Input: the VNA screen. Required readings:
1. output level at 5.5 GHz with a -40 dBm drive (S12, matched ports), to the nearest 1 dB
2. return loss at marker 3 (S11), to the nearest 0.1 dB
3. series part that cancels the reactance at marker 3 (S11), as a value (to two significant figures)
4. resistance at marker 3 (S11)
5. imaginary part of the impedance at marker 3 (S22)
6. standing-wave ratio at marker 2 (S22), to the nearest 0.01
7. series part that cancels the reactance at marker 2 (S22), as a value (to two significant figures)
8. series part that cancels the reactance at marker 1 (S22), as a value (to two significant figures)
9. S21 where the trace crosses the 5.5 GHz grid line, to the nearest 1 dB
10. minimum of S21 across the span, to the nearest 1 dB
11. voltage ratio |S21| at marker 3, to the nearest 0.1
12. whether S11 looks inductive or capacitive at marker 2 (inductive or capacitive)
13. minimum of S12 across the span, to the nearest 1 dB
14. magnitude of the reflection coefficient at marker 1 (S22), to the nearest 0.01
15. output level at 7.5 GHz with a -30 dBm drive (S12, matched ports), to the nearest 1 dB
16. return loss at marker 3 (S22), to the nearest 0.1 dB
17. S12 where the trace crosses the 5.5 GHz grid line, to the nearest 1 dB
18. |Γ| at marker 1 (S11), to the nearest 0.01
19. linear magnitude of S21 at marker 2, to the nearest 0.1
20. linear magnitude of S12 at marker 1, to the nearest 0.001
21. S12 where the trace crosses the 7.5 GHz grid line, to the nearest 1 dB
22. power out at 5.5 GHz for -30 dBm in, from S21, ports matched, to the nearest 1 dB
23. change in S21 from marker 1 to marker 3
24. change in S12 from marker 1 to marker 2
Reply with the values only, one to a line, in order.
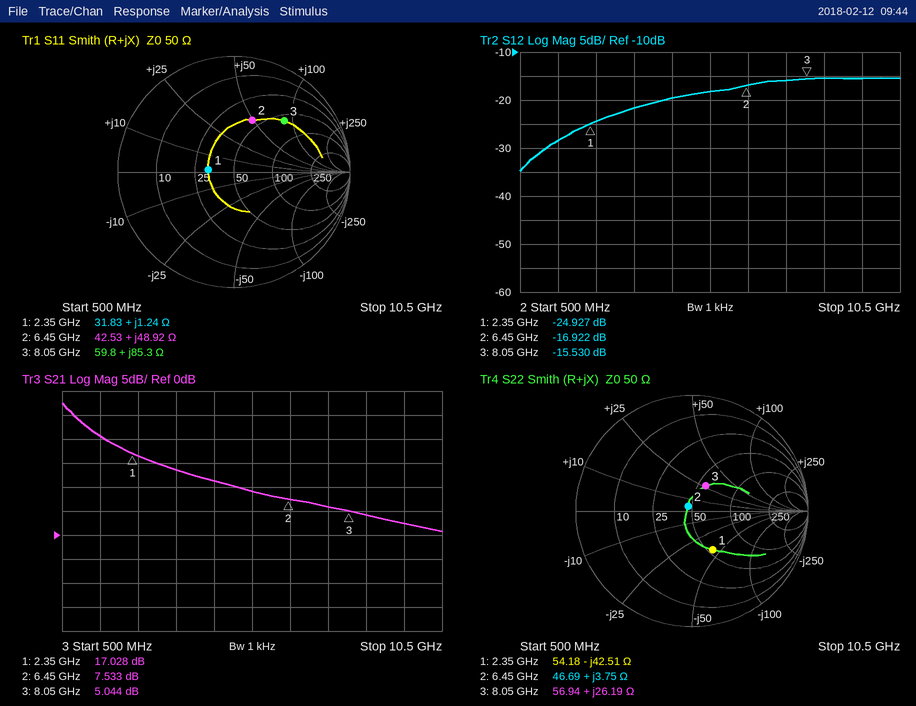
-58 dBm
4.2 dB
230 fF
59.8 Ω
+26.19 Ω
1.11
6.6 pF
2.9 nH
9 dB
1 dB
1.8
inductive
-35 dB
0.38
-46 dBm
12.2 dB
-18 dB
0.22
2.4
0.057
-16 dB
-21 dBm
-11.984 dB
8.005 dB
